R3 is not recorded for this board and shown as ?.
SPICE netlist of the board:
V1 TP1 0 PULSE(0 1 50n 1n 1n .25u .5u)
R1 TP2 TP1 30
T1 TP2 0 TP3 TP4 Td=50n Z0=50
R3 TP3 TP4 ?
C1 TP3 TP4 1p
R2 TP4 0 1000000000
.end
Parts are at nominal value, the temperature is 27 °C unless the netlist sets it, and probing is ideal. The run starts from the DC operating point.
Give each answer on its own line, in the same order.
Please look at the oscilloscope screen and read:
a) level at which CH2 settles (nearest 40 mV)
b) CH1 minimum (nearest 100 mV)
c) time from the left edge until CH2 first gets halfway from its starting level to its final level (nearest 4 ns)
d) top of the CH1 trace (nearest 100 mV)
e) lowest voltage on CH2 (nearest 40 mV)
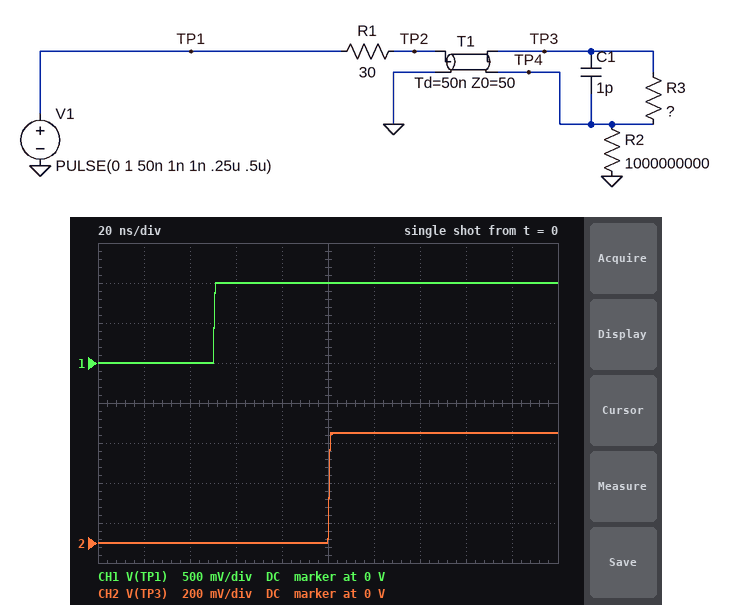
560 mV
0 V
100 ns
1.0 V
0 V
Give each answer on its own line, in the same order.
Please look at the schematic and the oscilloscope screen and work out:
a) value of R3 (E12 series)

39 Ω
